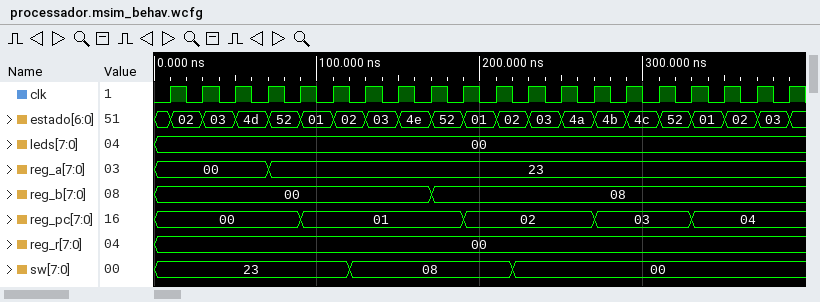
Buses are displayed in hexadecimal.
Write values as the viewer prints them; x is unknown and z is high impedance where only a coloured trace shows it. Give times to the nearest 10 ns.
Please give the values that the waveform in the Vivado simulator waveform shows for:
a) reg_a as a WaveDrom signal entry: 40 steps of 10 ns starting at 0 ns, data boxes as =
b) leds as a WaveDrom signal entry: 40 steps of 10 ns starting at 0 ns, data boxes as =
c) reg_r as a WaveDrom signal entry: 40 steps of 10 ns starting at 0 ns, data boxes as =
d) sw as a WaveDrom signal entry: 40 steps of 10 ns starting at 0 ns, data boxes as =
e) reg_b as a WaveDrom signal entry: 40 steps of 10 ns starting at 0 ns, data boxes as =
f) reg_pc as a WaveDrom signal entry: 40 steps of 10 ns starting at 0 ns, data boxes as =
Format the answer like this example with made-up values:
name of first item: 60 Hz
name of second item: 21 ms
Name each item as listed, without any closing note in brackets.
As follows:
reg_a as a WaveDrom signal entry: 40 steps of 10 ns starting at 0 ns, data boxes as =: {name: 'reg_a', wave: '=......=................................', data: '00 23'}
leds as a WaveDrom signal entry: 40 steps of 10 ns starting at 0 ns, data boxes as =: {name: 'leds', wave: '=.......................................', data: '00'}
reg_r as a WaveDrom signal entry: 40 steps of 10 ns starting at 0 ns, data boxes as =: {name: 'reg_r', wave: '=.......................................', data: '00'}
sw as a WaveDrom signal entry: 40 steps of 10 ns starting at 0 ns, data boxes as =: {name: 'sw', wave: '=...........=.........=.................', data: '23 08 00'}
reg_b as a WaveDrom signal entry: 40 steps of 10 ns starting at 0 ns, data boxes as =: {name: 'reg_b', wave: '=................=......................', data: '00 08'}
reg_pc as a WaveDrom signal entry: 40 steps of 10 ns starting at 0 ns, data boxes as =: {name: 'reg_pc', wave: '=........=.........=.......=.....=......', data: '00 01 02 03 04'}
